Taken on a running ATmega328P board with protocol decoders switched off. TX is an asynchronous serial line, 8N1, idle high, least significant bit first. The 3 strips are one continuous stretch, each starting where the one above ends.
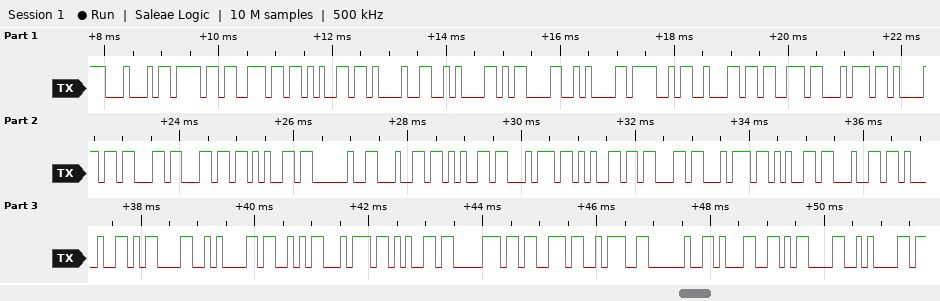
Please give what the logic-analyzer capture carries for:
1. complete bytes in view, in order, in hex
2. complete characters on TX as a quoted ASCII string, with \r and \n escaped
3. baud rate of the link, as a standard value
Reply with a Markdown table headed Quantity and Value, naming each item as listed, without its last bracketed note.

| Quantity | Value |
|---|---|
| complete bytes in view, in order, in hex | 44 6F 6E 65 21 0A 0D 0A 4F 62 73 74 61 63 6C 65 20 64 65 74 65 63 74 65 64 21 0D 0A 53 74 65 70 73 3A 20 31 0D 0A |
| complete characters on TX as a quoted ASCII string, with \r and \n escaped | "Done!\n\r\nObstacle detected!\r\nSteps: 1\r\n" |
| baud rate of the link, as a standard value | 9600 baud |
